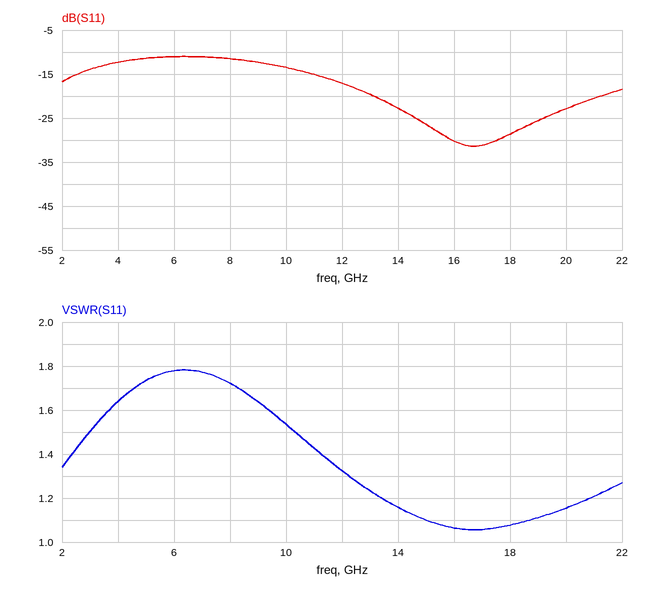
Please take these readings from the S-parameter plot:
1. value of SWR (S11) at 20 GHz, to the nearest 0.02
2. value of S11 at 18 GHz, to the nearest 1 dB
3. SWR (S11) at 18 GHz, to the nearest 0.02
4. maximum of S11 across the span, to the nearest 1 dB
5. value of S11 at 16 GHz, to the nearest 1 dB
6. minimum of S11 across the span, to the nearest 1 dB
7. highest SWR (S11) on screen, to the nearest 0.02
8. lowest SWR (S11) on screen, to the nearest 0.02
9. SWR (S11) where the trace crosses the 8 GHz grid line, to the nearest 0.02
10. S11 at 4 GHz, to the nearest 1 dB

1.16
-29 dB
1.08
-11 dB
-30 dB
-31 dB
1.78
1.06
1.72
-12 dB
